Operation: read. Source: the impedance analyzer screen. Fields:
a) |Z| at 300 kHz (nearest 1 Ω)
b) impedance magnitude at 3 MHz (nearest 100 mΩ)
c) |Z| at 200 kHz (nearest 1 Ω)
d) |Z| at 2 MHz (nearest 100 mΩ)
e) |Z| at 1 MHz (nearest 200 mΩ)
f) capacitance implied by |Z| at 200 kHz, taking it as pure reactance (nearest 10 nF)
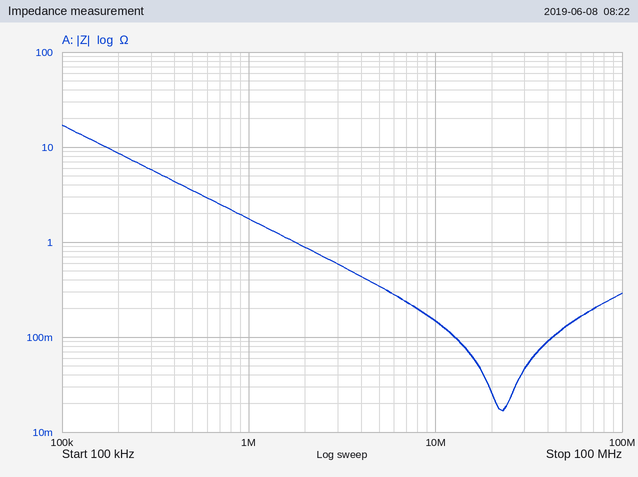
6 Ω
600 mΩ
9 Ω
900 mΩ
1.8 Ω
90 nF
